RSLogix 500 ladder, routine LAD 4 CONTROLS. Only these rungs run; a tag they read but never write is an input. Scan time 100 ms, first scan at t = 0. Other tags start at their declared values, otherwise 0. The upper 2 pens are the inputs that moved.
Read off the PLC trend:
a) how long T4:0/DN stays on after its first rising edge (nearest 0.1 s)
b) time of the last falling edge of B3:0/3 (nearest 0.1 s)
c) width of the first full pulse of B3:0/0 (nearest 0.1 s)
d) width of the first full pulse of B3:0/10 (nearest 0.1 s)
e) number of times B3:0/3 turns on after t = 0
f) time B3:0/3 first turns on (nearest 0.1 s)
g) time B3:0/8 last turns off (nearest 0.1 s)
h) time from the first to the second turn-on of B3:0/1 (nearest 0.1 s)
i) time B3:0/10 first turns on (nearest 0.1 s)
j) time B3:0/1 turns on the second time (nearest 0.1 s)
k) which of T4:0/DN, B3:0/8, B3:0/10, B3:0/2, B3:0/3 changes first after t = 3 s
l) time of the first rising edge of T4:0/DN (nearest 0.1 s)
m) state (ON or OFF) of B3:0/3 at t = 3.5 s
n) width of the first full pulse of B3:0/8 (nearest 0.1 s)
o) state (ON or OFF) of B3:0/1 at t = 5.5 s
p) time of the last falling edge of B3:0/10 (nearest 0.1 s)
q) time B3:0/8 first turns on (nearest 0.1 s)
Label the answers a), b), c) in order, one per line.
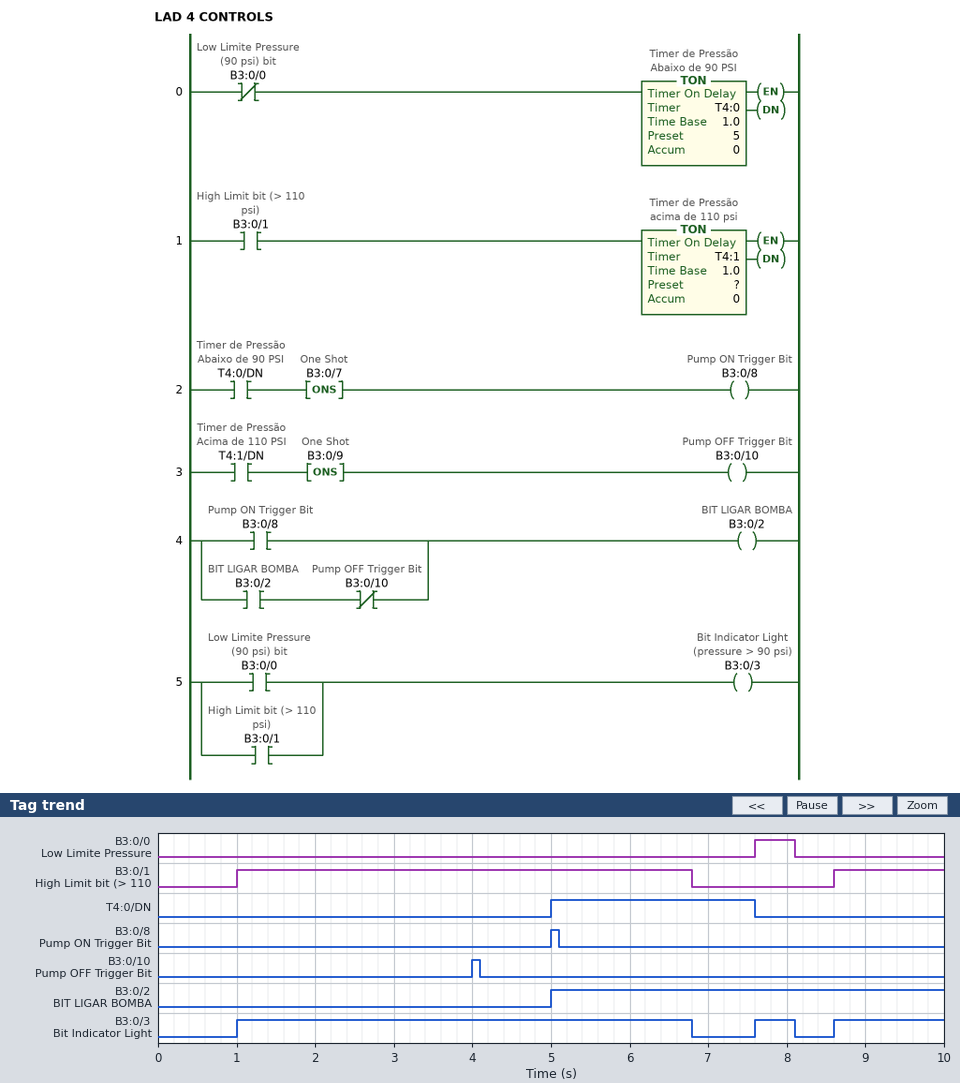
a) 2.6 s
b) 8.1 s
c) 0.5 s
d) 0.1 s
e) 3
f) 1.0 s
g) 5.1 s
h) 7.6 s
i) 4.0 s
j) 8.6 s
k) B3:0/10
l) 5.0 s
m) ON
n) 0.1 s
o) ON
p) 4.1 s
q) 5.0 s
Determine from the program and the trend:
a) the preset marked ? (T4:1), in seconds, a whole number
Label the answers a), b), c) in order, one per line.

a) 3 s
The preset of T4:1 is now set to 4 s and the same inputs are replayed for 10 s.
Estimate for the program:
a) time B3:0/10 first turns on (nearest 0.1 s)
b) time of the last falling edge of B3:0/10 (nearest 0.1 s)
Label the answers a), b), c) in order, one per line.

a) 5.0 s
b) 5.1 s
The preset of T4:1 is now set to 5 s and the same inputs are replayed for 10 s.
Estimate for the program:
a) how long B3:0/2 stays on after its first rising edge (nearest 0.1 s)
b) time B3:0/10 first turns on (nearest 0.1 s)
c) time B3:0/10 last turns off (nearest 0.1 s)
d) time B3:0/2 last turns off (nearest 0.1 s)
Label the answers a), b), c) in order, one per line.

a) 1.0 s
b) 6.0 s
c) 6.1 s
d) 6.0 s
